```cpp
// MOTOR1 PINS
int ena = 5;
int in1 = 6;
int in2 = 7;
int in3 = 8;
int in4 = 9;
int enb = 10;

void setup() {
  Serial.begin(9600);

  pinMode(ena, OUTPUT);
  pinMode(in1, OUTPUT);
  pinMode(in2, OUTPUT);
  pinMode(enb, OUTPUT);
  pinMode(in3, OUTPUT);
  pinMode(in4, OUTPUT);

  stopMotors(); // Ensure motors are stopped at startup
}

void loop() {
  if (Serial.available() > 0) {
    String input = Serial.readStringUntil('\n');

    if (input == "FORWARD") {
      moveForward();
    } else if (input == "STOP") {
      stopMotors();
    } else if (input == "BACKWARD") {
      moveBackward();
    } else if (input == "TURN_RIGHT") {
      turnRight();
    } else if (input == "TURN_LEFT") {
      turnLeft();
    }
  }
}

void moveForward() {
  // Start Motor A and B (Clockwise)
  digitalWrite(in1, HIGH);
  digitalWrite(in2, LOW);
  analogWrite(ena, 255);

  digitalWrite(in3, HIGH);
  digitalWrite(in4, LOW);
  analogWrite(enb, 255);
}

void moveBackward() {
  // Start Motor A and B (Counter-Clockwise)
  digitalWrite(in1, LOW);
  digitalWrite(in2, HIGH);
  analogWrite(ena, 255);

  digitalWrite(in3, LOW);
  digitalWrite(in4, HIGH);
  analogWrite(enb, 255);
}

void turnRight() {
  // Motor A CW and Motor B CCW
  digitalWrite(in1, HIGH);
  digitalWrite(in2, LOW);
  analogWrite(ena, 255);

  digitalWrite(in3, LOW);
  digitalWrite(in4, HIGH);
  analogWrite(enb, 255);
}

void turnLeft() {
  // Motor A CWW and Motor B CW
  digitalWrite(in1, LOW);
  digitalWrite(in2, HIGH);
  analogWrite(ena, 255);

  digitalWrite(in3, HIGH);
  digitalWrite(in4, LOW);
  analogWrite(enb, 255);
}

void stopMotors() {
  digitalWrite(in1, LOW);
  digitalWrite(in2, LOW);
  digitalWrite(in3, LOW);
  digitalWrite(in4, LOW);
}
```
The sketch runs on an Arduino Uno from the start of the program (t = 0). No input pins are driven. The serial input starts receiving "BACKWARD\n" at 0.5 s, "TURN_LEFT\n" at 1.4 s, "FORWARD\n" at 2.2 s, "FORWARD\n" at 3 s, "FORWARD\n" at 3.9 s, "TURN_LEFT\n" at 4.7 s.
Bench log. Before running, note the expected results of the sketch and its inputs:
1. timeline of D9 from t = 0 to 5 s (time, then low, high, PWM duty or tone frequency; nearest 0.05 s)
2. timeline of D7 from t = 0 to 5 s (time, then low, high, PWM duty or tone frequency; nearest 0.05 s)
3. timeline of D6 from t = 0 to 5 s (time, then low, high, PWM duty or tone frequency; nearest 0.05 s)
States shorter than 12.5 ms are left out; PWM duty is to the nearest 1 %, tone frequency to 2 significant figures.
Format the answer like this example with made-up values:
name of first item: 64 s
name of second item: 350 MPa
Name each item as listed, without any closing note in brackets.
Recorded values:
timeline of D9 from t = 0 to 5 s: 0 s low; 0.5 s high; 1.4 s low
timeline of D7 from t = 0 to 5 s: 0 s low; 0.5 s high; 2.2 s low; 4.7 s high
timeline of D6 from t = 0 to 5 s: 0 s low; 2.2 s high; 4.7 s low
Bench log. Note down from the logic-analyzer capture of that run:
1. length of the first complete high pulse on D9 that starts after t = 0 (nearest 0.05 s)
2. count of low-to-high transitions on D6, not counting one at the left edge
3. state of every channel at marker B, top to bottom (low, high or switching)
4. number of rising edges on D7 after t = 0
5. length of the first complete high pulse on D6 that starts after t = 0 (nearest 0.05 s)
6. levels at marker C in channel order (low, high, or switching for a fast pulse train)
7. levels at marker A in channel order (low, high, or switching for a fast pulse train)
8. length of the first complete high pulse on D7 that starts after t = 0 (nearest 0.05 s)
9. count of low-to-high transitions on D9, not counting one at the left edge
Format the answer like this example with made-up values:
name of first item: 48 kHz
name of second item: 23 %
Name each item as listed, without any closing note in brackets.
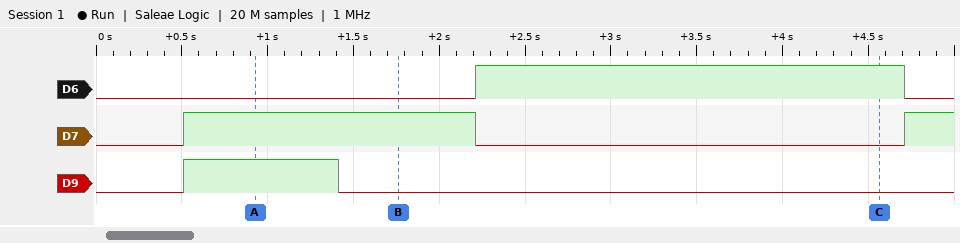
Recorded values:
length of the first complete high pulse on D9 that starts after t = 0: 0.90 s
count of low-to-high transitions on D6, not counting one at the left edge: 1
state of every channel at marker B, top to bottom: D6 low, D7 high, D9 low
number of rising edges on D7 after t = 0: 2
length of the first complete high pulse on D6 that starts after t = 0: 2.50 s
levels at marker C in channel order: D6 high, D7 low, D9 low
levels at marker A in channel order: D6 low, D7 high, D9 high
length of the first complete high pulse on D7 that starts after t = 0: 1.70 s
count of low-to-high transitions on D9, not counting one at the left edge: 1
